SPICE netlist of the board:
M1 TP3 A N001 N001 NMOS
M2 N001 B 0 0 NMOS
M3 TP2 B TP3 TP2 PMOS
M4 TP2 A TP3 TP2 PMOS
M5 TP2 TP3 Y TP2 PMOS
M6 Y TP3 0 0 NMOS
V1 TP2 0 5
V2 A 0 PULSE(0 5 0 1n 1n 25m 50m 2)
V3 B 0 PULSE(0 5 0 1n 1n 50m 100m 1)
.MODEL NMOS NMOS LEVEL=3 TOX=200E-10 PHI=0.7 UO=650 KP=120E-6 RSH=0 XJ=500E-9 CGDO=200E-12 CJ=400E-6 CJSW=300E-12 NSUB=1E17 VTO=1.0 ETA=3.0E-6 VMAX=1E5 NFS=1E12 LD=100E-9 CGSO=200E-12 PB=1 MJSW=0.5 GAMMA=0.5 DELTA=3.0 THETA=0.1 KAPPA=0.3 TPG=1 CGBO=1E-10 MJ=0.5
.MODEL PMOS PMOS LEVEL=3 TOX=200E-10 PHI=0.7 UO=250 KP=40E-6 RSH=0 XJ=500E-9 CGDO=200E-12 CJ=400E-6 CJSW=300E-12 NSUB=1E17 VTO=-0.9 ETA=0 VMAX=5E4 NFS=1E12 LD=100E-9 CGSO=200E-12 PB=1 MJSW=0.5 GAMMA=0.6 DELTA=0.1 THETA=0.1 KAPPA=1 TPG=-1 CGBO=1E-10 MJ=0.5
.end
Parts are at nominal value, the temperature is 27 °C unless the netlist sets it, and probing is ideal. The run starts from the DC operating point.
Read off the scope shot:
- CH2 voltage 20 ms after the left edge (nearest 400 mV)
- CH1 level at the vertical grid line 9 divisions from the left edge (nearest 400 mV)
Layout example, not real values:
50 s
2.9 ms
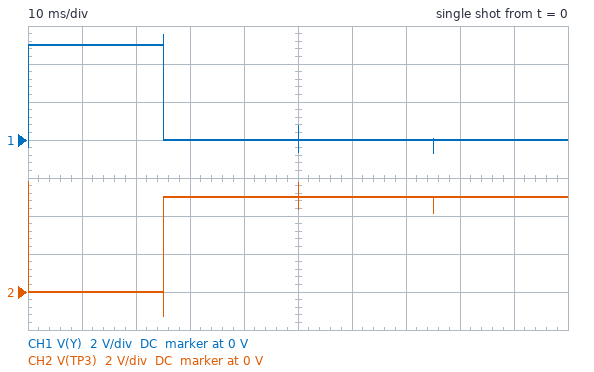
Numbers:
0 V
0 V
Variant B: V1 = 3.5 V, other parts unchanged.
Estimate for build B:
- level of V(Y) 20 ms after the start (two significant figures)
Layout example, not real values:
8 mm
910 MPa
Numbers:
3.5 V
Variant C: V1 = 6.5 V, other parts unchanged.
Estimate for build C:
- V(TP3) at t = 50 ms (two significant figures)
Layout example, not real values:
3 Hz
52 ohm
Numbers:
6.5 V
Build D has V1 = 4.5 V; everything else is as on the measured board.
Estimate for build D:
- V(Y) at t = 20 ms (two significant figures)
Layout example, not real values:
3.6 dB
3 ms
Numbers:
4.5 V
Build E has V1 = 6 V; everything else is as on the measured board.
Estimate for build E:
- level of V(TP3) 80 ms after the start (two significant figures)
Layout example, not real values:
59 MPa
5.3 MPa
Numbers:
6.0 V
